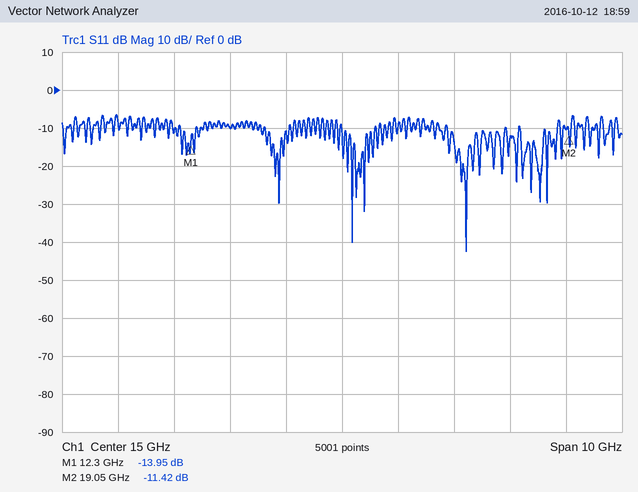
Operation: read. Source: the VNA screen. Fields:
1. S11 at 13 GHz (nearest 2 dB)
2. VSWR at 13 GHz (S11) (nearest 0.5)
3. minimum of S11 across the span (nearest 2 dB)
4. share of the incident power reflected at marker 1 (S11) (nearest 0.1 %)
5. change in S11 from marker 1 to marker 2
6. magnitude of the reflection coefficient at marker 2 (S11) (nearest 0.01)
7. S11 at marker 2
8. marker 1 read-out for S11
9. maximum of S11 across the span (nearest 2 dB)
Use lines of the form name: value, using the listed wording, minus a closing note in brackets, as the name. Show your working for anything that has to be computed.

S11 at 13 GHz: -10 dB
VSWR at 13 GHz (S11): |Γ| = 10^(-10/20) = 0.3162; VSWR = (1 + 0.3162)/(1 − 0.3162) ≈ 1.92, so 2.0 to the nearest 0.5
minimum of S11 across the span: -42 dB
share of the incident power reflected at marker 1 (S11): 10^(-13.95/10) ≈ 4.0 %
change in S11 from marker 1 to marker 2: -11.42 − (-13.95) = 2.53 dB
magnitude of the reflection coefficient at marker 2 (S11): 10^(-11.42/20) ≈ 0.27
S11 at marker 2: -11.42 dB
marker 1 read-out for S11: -13.95 dB
maximum of S11 across the span: -6 dB
